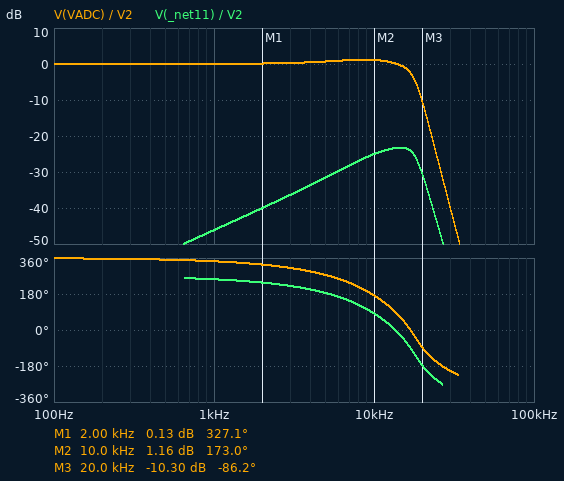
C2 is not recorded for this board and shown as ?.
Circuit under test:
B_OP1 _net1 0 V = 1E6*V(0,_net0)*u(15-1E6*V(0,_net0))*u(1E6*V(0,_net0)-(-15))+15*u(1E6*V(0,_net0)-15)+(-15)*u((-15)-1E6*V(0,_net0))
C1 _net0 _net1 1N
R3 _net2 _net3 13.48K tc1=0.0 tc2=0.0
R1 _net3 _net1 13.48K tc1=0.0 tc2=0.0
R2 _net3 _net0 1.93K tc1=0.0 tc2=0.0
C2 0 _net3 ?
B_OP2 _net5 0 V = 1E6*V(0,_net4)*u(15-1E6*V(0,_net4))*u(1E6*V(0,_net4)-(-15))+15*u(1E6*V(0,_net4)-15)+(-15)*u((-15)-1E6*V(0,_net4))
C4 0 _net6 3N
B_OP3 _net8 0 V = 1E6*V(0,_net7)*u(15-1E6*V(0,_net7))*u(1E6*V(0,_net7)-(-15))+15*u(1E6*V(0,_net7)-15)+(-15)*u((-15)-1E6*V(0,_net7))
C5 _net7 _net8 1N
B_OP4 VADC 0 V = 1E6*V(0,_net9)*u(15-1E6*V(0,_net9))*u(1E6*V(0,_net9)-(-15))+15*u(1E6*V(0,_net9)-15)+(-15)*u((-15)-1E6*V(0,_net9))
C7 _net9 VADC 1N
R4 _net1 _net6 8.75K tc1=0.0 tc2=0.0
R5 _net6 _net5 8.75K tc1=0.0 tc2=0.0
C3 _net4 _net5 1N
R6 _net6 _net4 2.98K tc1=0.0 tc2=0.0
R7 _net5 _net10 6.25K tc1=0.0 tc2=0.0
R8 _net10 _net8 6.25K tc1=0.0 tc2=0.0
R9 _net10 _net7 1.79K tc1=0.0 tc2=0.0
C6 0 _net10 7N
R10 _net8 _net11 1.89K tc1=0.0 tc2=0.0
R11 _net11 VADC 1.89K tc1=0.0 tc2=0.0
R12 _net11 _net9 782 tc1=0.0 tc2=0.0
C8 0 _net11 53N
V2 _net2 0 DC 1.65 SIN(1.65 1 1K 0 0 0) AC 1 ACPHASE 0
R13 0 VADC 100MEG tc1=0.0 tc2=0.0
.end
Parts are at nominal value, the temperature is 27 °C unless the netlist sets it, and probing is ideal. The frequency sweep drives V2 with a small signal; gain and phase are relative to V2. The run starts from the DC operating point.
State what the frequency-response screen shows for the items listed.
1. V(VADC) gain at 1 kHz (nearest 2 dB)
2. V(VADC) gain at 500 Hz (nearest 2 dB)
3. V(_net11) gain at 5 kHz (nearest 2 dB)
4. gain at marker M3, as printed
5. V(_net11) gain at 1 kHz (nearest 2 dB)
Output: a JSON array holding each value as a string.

["0 dB", "0 dB", "-32 dB", "-10.30 dB", "-46 dB"]
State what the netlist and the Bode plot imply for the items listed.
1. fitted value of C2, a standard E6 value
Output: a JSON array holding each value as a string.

["6.8 nF"]
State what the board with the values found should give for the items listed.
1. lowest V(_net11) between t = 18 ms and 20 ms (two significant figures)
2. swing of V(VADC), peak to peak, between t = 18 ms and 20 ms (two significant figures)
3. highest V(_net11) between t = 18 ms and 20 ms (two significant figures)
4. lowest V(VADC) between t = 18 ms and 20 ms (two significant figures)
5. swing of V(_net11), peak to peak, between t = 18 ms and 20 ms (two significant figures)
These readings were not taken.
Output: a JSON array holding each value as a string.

["-4.9 mV", "2.0 V", "4.9 mV", "650 mV", "9.9 mV"]
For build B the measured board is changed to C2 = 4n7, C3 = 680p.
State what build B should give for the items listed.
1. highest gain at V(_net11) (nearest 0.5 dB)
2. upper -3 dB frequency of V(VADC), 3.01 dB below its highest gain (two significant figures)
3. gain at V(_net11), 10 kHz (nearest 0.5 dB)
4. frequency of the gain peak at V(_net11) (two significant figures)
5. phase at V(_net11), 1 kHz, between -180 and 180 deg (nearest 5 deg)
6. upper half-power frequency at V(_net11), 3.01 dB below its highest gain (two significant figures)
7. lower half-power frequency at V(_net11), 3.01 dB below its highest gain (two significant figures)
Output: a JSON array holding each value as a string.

["-20.0 dB", "18 kHz", "-24.5 dB", "16 kHz", "-105 deg", "19 kHz", "11 kHz"]
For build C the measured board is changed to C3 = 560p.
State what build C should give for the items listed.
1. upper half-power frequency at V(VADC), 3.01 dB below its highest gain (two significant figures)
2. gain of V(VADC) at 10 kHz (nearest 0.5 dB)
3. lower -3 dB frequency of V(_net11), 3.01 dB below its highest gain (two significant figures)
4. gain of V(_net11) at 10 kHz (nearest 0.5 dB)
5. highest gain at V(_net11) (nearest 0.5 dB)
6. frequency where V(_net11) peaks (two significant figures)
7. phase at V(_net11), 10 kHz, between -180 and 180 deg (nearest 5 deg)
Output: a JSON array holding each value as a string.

["18 kHz", "2.5 dB", "11 kHz", "-23.5 dB", "-20.0 dB", "16 kHz", "105 deg"]
